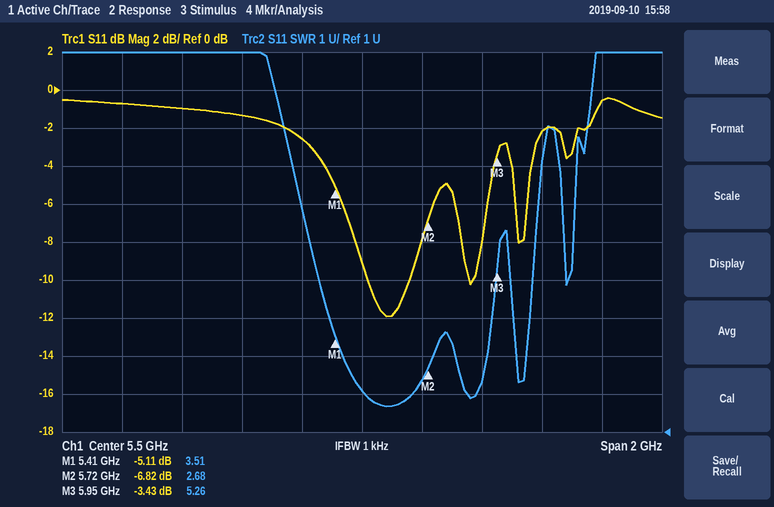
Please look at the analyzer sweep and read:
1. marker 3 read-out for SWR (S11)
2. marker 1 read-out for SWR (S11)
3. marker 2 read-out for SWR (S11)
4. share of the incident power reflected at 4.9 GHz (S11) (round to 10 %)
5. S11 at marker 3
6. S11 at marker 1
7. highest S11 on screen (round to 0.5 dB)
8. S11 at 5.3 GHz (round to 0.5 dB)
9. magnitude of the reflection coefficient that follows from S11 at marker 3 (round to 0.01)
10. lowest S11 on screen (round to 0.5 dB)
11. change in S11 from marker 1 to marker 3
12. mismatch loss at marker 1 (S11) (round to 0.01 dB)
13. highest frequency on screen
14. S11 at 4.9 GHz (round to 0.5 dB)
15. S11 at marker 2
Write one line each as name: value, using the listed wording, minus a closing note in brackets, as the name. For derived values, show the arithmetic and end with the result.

marker 3 read-out for SWR: 5.26
marker 1 read-out for SWR: 3.51
marker 2 read-out for SWR: 2.68
share of the incident power reflected at 4.9 GHz (S11): 10^(-1/10) ≈ 79.4 %, so 80 % to the nearest 10 %
S11 at marker 3: -3.43 dB
S11 at marker 1: -5.11 dB
highest S11 on screen: -0.5 dB
S11 at 5.3 GHz: -2.5 dB
magnitude of the reflection coefficient that follows from S11 at marker 3: 10^(-3.43/20) ≈ 0.67
lowest S11 on screen: -12.0 dB
change in S11 from marker 1 to marker 3: -3.43 − (-5.11) = 1.68 dB
mismatch loss at marker 1 (S11): −10 log10(1 − 10^(-5.11/10)) ≈ 1.60 dB
highest frequency on screen: 6.5 GHz
S11 at 4.9 GHz: -1.0 dB
S11 at marker 2: -6.82 dB
